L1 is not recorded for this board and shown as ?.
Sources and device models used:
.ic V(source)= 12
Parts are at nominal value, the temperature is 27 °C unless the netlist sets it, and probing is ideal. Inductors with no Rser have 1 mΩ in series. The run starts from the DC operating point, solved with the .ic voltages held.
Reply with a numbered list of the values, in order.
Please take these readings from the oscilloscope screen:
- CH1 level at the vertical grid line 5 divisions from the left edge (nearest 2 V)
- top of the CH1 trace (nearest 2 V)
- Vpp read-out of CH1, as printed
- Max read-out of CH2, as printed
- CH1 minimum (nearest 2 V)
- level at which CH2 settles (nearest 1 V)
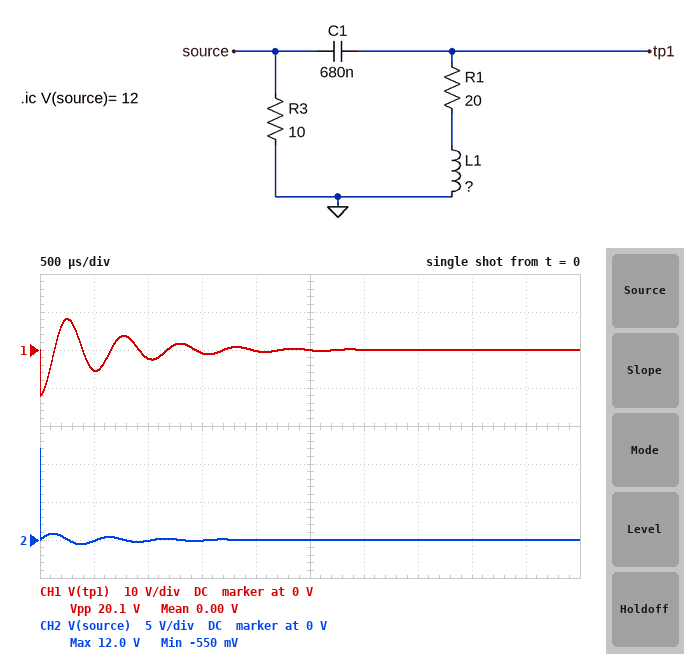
1. 0 V
2. 8 V
3. 20.1 V
4. 12.0 V
5. -12 V
6. 0 V
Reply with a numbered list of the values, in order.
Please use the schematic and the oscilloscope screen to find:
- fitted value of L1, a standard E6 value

1. 10 mH
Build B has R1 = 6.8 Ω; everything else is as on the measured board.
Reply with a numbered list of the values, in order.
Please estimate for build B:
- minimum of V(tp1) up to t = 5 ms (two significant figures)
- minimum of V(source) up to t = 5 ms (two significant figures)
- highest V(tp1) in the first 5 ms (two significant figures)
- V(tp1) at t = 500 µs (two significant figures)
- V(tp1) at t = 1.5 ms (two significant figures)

1. -12 V
2. -720 mV
3. 9.7 V
4. -7.7 V
5. -2.6 V
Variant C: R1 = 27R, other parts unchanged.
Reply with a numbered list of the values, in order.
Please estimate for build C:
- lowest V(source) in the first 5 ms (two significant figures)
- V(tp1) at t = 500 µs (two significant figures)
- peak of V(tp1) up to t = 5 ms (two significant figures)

1. -490 mV
2. -4.5 V
3. 7.4 V
